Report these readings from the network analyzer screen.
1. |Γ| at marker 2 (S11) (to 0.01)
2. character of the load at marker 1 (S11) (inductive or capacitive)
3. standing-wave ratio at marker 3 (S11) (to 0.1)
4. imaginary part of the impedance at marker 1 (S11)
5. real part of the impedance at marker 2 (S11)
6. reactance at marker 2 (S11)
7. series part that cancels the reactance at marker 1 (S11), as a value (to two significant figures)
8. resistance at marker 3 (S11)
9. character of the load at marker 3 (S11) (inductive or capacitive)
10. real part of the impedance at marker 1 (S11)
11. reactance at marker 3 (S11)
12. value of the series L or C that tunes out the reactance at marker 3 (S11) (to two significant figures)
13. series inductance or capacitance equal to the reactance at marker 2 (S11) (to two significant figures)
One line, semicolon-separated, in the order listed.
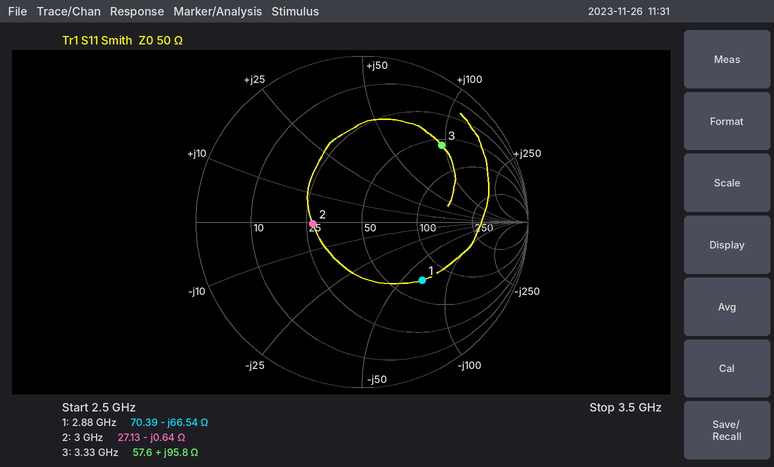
0.30; capacitive; 5.0; -66.54 Ω; 27.13 Ω; -0.64 Ω; 3.7 nH; 57.6 Ω; inductive; 70.39 Ω; +95.8 Ω; 500 fF; 83 pF
